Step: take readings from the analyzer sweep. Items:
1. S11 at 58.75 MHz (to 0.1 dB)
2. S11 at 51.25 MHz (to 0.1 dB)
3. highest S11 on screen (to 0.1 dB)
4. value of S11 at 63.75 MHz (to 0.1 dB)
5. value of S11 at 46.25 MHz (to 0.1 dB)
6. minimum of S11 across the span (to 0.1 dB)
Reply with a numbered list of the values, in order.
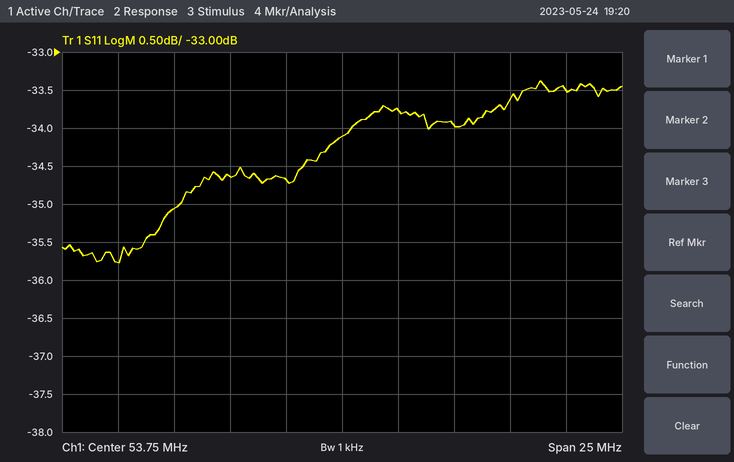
1. -34.0 dB
2. -34.7 dB
3. -33.4 dB
4. -33.5 dB
5. -35.1 dB
6. -35.8 dB
